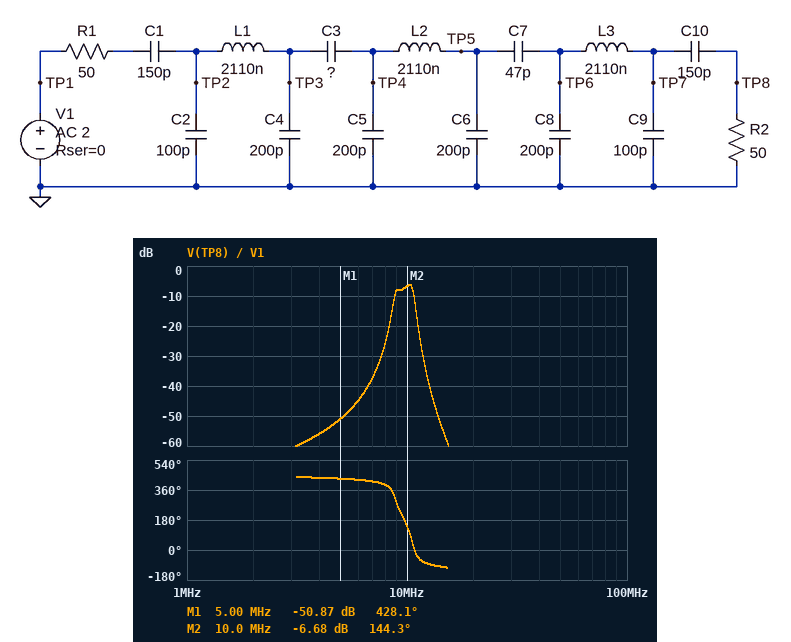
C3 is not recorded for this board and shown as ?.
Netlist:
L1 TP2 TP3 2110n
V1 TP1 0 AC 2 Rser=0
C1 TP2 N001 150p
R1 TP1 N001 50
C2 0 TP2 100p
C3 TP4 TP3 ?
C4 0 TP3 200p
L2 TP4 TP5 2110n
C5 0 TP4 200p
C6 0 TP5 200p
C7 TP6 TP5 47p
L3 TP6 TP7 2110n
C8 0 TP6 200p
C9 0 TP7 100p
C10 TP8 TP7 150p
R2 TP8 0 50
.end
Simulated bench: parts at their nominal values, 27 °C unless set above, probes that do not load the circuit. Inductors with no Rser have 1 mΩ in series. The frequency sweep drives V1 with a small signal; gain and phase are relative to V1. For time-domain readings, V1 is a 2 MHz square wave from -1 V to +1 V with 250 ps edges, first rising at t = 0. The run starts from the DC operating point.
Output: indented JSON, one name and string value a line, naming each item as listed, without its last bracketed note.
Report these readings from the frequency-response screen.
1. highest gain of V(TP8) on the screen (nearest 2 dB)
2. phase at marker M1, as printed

{
  "highest gain of V(TP8) on the screen": "-6 dB",
  "phase at marker M1, as printed": "428.1 deg"
}
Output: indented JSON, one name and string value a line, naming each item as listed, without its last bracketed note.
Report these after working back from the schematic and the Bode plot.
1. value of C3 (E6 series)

{
  "value of C3": "100 pF"
}
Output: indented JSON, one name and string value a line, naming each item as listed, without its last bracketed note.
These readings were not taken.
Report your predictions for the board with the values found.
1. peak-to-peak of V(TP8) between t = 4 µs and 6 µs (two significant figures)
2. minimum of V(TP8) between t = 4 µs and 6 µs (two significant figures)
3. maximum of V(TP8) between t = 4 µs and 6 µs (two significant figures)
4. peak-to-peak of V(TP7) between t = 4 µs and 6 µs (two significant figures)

{
  "peak-to-peak of V(TP8) between t = 4 µs and 6 µs": "240 mV",
  "minimum of V(TP8) between t = 4 µs and 6 µs": "-120 mV",
  "maximum of V(TP8) between t = 4 µs and 6 µs": "120 mV",
  "peak-to-peak of V(TP7) between t = 4 µs and 6 µs": "580 mV"
}
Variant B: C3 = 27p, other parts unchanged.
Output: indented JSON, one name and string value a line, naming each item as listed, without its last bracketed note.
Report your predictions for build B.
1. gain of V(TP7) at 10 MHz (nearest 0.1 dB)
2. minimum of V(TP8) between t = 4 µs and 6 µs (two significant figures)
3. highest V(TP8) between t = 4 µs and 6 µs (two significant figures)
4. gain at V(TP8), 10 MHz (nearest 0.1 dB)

{
  "gain of V(TP7) at 10 MHz": "0.2 dB",
  "minimum of V(TP8) between t = 4 µs and 6 µs": "-110 mV",
  "highest V(TP8) between t = 4 µs and 6 µs": "110 mV",
  "gain at V(TP8), 10 MHz": "-7.2 dB"
}
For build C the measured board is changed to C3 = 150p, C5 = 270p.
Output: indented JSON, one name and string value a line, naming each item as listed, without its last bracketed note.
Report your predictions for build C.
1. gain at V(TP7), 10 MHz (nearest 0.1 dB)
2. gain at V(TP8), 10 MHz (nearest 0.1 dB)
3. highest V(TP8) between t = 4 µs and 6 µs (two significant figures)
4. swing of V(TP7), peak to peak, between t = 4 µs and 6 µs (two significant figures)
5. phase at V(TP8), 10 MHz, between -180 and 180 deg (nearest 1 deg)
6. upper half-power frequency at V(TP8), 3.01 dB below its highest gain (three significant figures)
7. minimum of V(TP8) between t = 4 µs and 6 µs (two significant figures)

{
  "gain at V(TP7), 10 MHz": "0.2 dB",
  "gain at V(TP8), 10 MHz": "-7.2 dB",
  "highest V(TP8) between t = 4 µs and 6 µs": "110 mV",
  "swing of V(TP7), peak to peak, between t = 4 µs and 6 µs": "550 mV",
  "phase at V(TP8), 10 MHz, between -180 and 180 deg": "102 deg",
  "upper half-power frequency at V(TP8), 3.01 dB below its highest gain": "10.4 MHz",
  "minimum of V(TP8) between t = 4 µs and 6 µs": "-110 mV"
}
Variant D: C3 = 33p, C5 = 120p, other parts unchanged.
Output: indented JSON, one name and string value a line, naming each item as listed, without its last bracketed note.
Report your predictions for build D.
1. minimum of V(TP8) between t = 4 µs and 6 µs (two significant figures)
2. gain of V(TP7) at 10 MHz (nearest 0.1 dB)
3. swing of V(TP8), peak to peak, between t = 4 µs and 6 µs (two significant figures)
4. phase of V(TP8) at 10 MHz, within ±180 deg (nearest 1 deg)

{
  "minimum of V(TP8) between t = 4 µs and 6 µs": "-64 mV",
  "gain of V(TP7) at 10 MHz": "-4.7 dB",
  "swing of V(TP8), peak to peak, between t = 4 µs and 6 µs": "130 mV",
  "phase of V(TP8) at 10 MHz, within ±180 deg": "-122 deg"
}
